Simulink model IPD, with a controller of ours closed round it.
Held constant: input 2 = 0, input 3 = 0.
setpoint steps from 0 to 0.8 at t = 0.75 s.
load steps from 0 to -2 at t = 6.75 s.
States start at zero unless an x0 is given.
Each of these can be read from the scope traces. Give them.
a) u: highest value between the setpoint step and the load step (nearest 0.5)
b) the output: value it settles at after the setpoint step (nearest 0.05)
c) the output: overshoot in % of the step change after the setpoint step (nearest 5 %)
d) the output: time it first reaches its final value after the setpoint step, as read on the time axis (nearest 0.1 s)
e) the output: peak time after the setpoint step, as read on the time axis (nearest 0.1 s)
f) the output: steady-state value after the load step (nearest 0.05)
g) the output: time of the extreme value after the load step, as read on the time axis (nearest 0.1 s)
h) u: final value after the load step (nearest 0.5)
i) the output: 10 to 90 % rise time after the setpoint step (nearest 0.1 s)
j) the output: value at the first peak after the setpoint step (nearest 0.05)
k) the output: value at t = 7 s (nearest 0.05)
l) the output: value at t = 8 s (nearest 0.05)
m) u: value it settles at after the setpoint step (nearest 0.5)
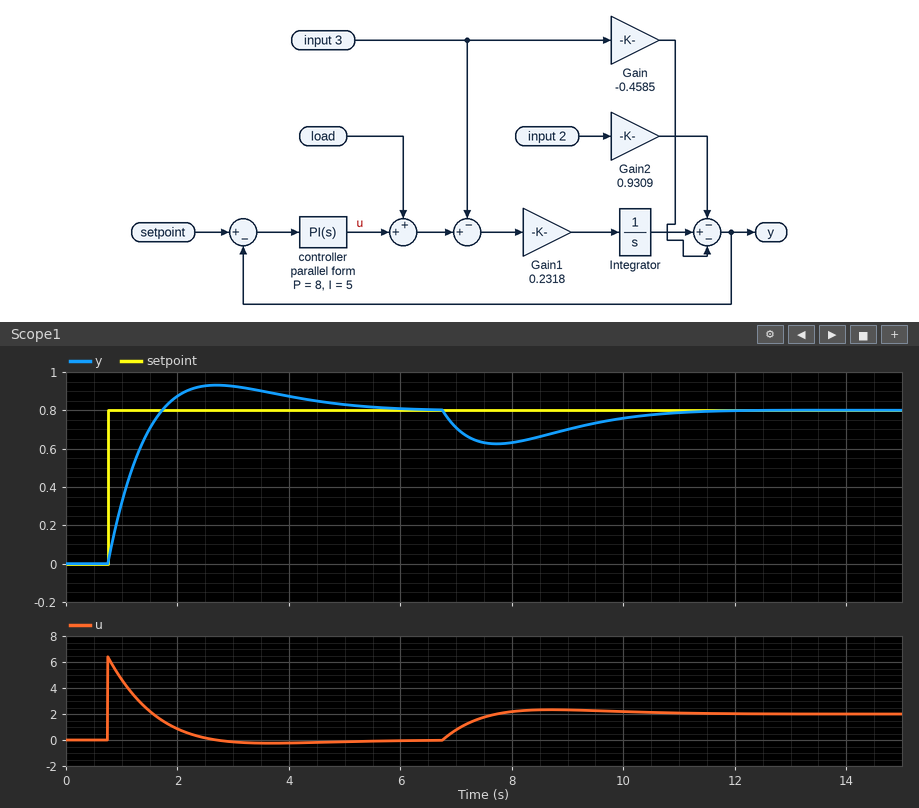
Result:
6.5
0.80
15 %
1.7 s
2.7 s
0.80
7.7 s
2.0
0.7 s
0.95
0.70
0.65
0.0
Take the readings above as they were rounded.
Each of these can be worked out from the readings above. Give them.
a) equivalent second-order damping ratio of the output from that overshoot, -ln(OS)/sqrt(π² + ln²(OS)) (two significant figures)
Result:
0.52
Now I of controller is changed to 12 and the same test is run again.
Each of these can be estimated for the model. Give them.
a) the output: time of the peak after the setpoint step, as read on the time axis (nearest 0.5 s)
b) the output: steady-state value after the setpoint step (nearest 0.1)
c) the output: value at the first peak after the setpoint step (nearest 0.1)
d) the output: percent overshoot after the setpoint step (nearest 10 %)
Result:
2.0 s
0.8
1.0
30 %
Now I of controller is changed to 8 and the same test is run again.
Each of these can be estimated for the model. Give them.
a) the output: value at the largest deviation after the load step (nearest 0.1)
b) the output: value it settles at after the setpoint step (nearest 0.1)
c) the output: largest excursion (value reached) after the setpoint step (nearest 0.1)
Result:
0.6
0.8
1.0
